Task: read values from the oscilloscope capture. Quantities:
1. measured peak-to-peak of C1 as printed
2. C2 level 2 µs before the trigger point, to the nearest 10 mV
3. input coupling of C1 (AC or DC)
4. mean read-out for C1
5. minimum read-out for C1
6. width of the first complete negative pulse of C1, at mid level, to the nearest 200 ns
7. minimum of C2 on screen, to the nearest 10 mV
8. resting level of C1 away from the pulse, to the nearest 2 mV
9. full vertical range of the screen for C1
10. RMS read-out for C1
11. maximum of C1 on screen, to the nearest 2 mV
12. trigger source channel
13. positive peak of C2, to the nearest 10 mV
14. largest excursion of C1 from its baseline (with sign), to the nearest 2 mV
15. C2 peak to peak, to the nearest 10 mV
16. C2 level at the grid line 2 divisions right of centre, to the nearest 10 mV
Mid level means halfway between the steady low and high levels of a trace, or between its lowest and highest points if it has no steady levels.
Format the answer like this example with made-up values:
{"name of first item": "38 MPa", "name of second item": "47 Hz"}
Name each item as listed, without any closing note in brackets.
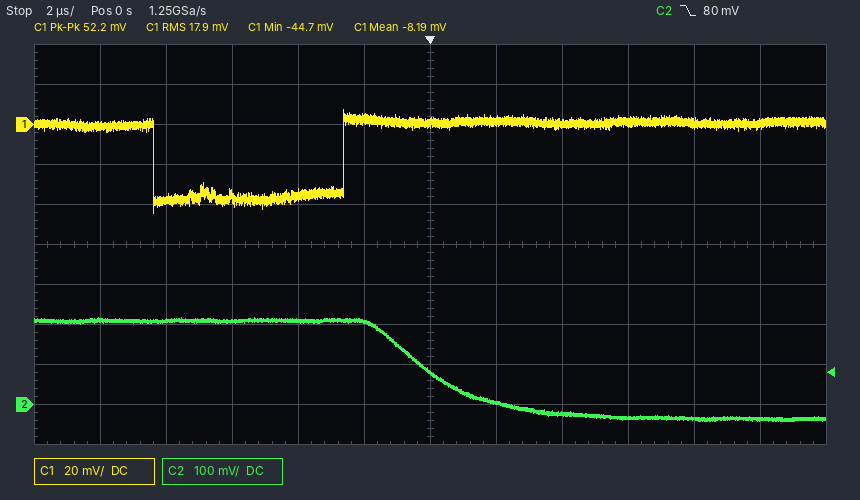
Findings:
{"measured peak-to-peak of C1 as printed": "52.2 mV", "C2 level 2 µs before the trigger point, to the nearest 10 mV": "210 mV", "input coupling of C1": "DC", "mean read-out for C1": "-8.19 mV", "minimum read-out for C1": "-44.7 mV", "width of the first complete negative pulse of C1, at mid level, to the nearest 200 ns": "5.8 µs", "minimum of C2 on screen, to the nearest 10 mV": "-40 mV", "resting level of C1 away from the pulse, to the nearest 2 mV": "0 mV", "full vertical range of the screen for C1": "200 mV", "RMS read-out for C1": "17.9 mV", "maximum of C1 on screen, to the nearest 2 mV": "8 mV", "trigger source channel": "C2", "positive peak of C2, to the nearest 10 mV": "220 mV", "largest excursion of C1 from its baseline (with sign), to the nearest 2 mV": "-46 mV", "C2 peak to peak, to the nearest 10 mV": "260 mV", "C2 level at the grid line 2 divisions right of centre, to the nearest 10 mV": "-20 mV"}
